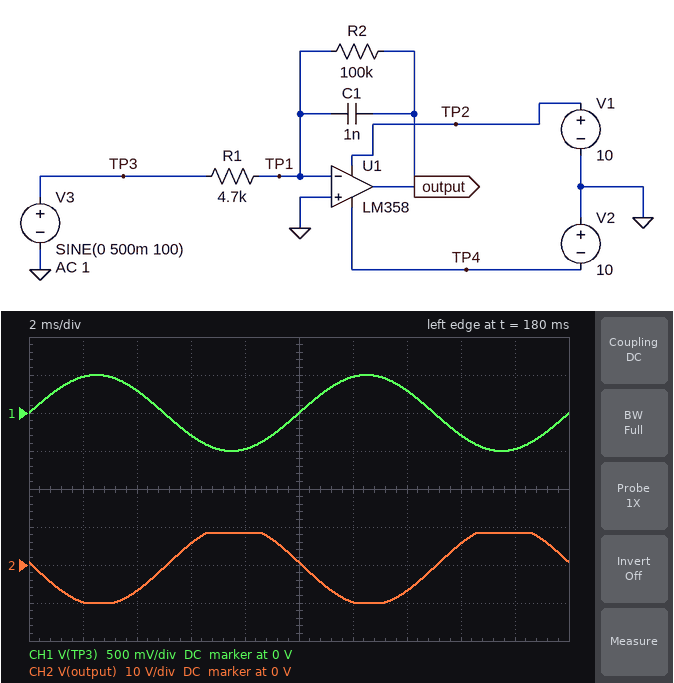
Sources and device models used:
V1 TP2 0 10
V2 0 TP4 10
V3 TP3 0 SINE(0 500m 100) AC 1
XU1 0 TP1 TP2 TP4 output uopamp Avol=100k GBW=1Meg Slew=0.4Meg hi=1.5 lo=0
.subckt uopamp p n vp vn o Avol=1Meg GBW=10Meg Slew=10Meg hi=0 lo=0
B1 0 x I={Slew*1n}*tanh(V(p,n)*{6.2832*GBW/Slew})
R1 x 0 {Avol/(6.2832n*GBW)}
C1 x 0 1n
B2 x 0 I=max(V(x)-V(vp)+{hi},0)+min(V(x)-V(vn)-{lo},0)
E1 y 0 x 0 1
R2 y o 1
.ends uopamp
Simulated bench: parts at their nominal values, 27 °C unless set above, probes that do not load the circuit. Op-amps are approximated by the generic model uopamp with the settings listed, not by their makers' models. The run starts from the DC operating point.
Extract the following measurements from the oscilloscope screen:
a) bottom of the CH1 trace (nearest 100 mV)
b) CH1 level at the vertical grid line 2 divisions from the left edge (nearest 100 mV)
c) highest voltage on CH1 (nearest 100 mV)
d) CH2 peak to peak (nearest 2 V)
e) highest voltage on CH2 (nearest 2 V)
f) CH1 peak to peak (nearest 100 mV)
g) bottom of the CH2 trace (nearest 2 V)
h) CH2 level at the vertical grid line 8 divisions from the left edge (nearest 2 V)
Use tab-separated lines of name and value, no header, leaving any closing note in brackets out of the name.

bottom of the CH1 trace	-500 mV
CH1 level at the vertical grid line 2 divisions from the left edge	300 mV
highest voltage on CH1	500 mV
CH2 peak to peak	18 V
highest voltage on CH2	8 V
CH1 peak to peak	1.0 V
bottom of the CH2 trace	-10 V
CH2 level at the vertical grid line 8 divisions from the left edge	6 V
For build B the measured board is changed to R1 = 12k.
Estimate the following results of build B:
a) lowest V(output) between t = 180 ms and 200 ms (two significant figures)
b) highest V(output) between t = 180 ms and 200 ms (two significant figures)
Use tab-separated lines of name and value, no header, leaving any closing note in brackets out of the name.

lowest V(output) between t = 180 ms and 200 ms	-4.2 V
highest V(output) between t = 180 ms and 200 ms	4.2 V
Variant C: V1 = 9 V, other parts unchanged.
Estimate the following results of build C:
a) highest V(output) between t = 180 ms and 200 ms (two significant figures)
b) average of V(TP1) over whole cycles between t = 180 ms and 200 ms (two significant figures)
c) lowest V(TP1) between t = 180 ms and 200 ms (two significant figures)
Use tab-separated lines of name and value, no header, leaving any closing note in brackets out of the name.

highest V(output) between t = 180 ms and 200 ms	7.5 V
average of V(TP1) over whole cycles between t = 180 ms and 200 ms	-21 mV
lowest V(TP1) between t = 180 ms and 200 ms	-140 mV
